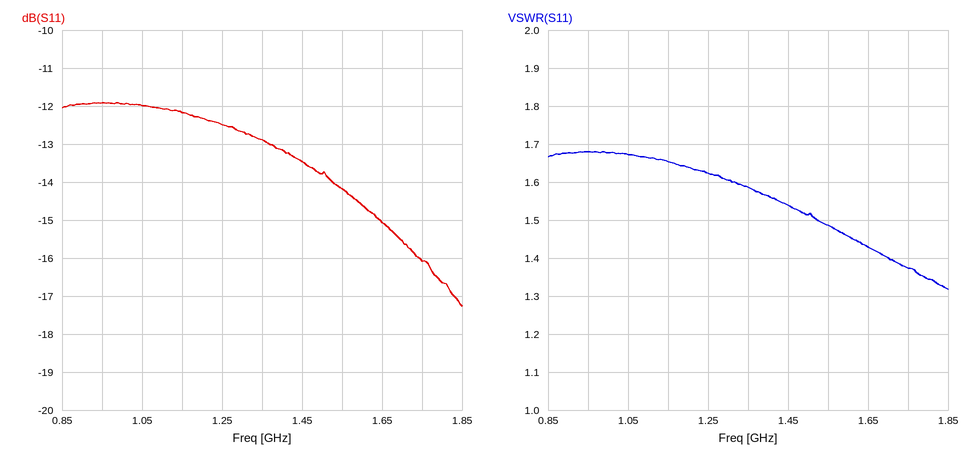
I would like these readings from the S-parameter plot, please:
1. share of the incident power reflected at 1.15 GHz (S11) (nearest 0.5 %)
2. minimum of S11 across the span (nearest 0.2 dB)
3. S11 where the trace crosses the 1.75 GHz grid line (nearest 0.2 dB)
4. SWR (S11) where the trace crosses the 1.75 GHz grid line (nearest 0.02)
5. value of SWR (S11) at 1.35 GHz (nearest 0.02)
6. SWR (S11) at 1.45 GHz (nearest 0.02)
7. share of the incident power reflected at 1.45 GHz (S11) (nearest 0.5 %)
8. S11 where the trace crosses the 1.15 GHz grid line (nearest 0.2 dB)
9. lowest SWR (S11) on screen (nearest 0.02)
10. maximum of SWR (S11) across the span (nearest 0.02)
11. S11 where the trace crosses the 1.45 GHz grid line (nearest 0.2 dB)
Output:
6.0 %
-17.2 dB
-16.0 dB
1.38
1.58
1.54
4.5 %
-12.2 dB
1.32
1.68
-13.4 dB
